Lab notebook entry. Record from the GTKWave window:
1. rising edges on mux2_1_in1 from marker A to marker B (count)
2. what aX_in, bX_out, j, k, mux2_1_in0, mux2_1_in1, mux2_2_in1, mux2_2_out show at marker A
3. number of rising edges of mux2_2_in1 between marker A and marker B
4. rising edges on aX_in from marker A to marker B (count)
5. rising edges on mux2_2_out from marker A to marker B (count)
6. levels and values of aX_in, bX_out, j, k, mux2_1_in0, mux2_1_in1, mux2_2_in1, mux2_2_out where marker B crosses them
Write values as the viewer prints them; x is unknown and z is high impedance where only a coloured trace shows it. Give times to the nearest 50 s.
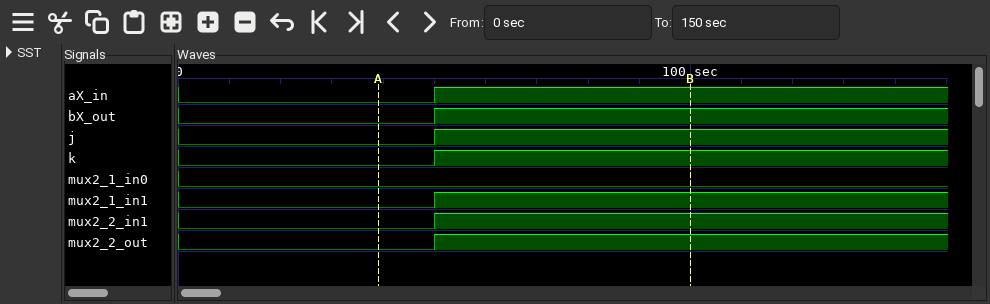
1
aX_in=0, bX_out=0, j=0, k=0, mux2_1_in0=0, mux2_1_in1=0, mux2_2_in1=0, mux2_2_out=0
1
1
1
aX_in=1, bX_out=1, j=1, k=1, mux2_1_in0=0, mux2_1_in1=1, mux2_2_in1=1, mux2_2_out=1
